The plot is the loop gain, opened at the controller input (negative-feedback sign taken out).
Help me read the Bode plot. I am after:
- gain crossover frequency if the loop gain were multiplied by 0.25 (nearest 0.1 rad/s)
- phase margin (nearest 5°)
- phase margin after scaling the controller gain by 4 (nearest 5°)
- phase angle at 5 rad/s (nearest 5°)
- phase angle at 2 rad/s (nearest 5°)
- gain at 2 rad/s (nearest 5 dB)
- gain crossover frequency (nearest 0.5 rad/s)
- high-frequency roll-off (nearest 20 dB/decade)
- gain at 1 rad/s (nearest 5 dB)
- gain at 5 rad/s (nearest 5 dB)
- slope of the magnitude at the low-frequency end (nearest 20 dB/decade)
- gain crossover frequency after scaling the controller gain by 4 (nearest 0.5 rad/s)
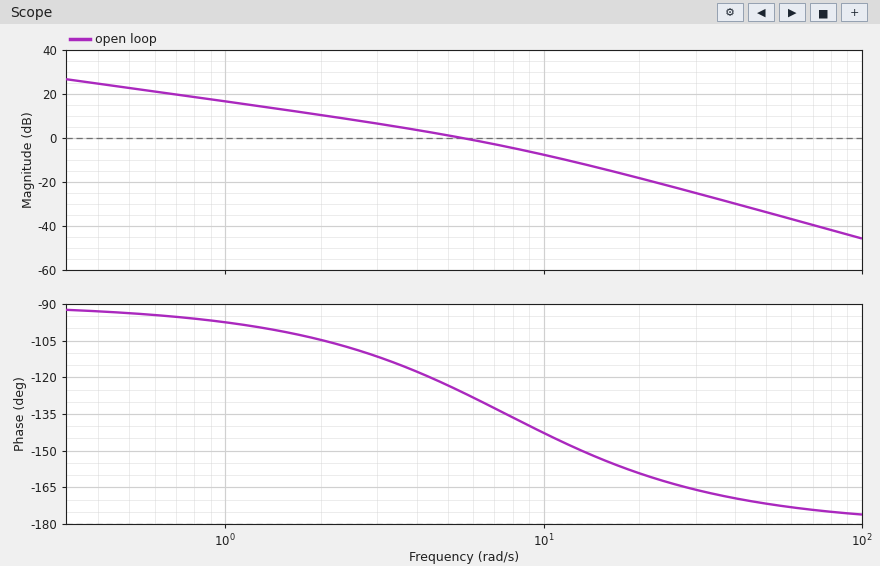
1.7 rad/s
55°
30°
-125°
-105°
10 dB
5.5 rad/s
-40 dB/decade
15 dB
0 dB
-20 dB/decade
13.5 rad/s
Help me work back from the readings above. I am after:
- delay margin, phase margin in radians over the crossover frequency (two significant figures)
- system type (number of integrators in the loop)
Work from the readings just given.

0.17 s
1
